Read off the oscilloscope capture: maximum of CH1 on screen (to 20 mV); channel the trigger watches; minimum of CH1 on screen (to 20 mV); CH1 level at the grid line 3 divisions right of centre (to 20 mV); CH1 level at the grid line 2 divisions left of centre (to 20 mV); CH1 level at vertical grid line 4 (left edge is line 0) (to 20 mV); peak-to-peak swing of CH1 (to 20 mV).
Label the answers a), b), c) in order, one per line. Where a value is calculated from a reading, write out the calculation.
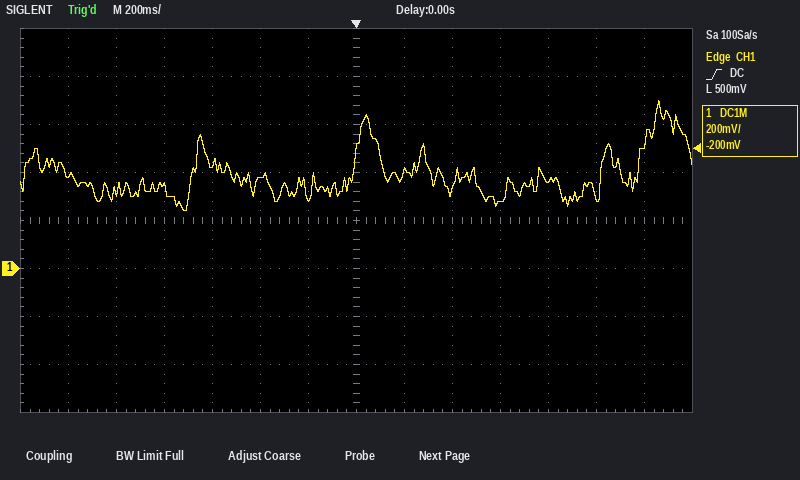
a) 700 mV
b) CH1
c) 240 mV
d) 280 mV
e) 380 mV
f) 440 mV
g) 700 mV − (240 mV) = 460 mV
